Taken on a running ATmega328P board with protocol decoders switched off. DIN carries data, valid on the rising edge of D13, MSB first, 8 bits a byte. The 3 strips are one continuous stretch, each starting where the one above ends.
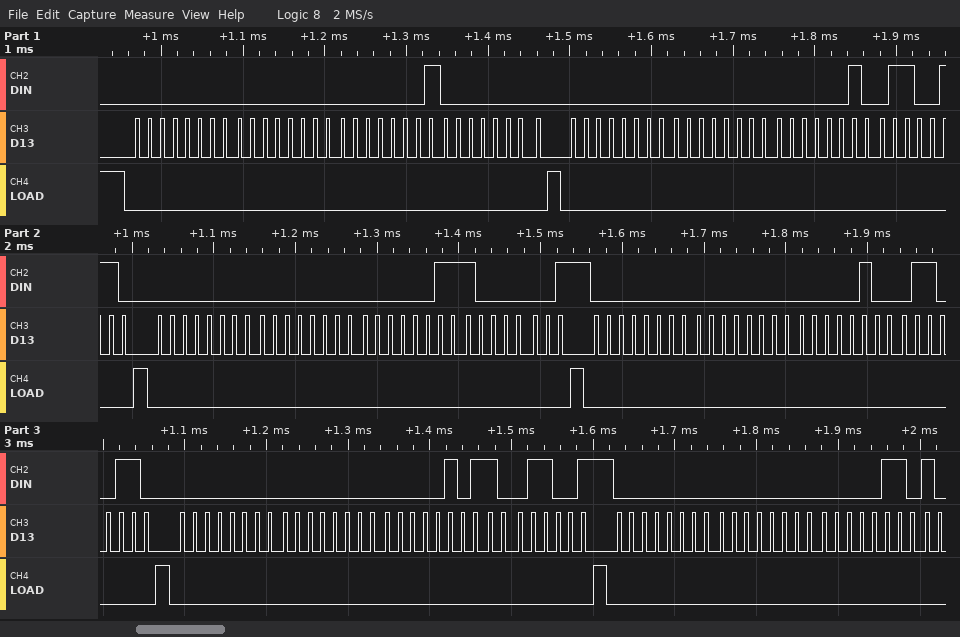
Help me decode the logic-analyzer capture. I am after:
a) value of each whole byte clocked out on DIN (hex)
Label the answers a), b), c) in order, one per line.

a) 00 00 01 00 00 00 02 66 00 00 03 81 00 00 04 66 00 00 05 99 00 00 06
